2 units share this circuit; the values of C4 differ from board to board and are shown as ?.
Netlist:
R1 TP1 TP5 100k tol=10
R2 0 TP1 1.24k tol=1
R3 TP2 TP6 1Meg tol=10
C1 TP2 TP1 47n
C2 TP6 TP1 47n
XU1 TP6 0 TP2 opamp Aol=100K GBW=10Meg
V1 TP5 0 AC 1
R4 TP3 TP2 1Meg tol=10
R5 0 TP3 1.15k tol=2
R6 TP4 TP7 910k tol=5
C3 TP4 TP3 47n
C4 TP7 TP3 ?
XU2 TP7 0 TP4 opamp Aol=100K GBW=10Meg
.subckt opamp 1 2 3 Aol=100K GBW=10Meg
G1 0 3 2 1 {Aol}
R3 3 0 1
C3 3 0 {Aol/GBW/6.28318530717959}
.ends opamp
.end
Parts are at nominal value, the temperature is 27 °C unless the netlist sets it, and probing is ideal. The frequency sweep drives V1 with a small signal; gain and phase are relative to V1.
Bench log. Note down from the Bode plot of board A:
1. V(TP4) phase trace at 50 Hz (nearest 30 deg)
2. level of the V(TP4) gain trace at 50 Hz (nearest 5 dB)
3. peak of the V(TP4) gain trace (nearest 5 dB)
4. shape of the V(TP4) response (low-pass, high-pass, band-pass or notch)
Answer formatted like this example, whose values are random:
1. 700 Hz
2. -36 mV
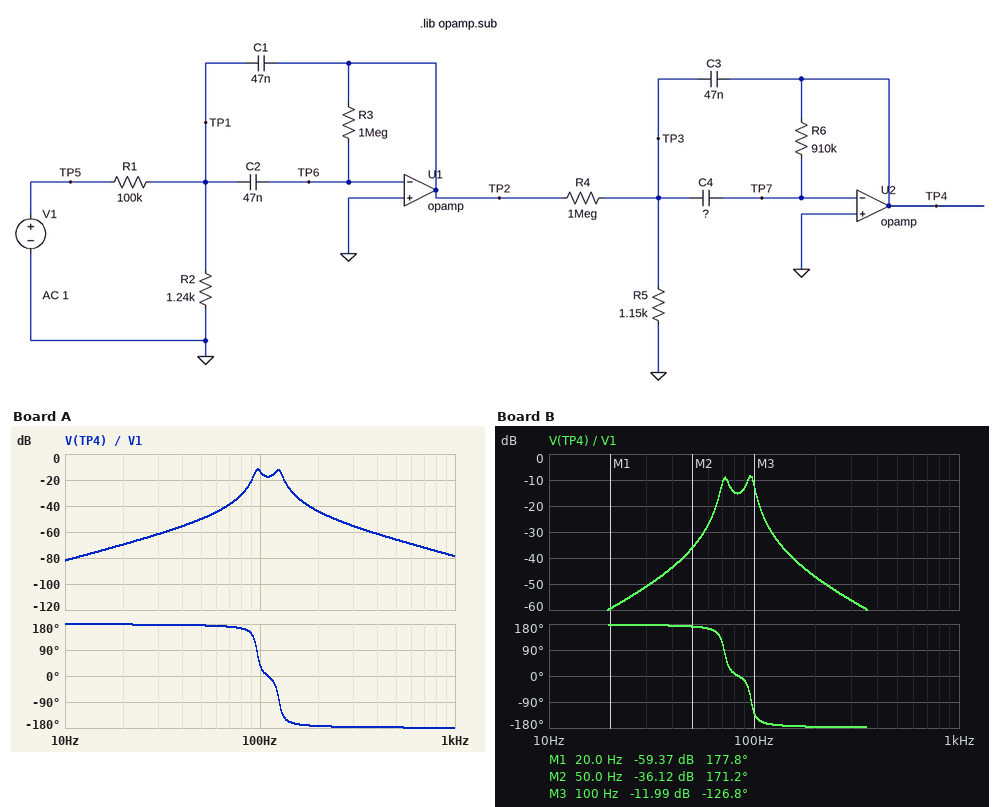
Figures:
1. 180 deg
2. -50 dB
3. -10 dB
4. band-pass
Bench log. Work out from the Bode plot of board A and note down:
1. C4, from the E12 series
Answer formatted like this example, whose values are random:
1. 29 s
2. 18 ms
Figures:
1. 33 nF
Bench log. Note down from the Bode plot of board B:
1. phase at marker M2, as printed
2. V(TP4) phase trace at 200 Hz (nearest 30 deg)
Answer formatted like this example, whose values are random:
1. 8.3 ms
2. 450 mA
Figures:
1. 171.2 deg
2. -180 deg
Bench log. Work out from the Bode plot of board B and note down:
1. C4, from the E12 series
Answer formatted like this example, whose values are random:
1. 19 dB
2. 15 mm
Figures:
1. 100 nF
